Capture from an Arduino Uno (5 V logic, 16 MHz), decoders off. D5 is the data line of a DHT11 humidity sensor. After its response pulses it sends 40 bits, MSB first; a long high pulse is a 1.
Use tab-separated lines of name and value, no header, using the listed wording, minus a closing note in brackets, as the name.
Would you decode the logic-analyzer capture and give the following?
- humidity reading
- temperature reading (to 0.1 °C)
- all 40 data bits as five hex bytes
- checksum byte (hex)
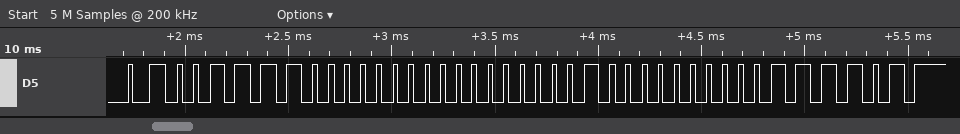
humidity reading	60 %
temperature reading	1.0 °C
all 40 data bits as five hex bytes	3C 00 01 00 3D
checksum byte	0x3D
